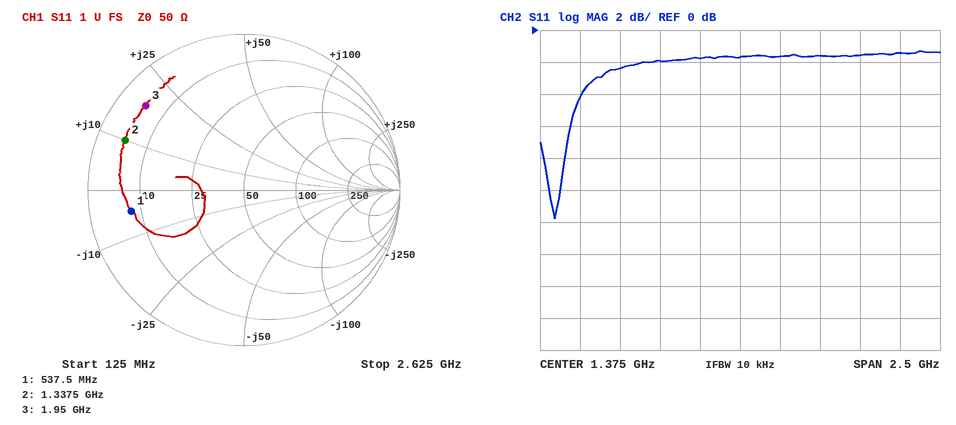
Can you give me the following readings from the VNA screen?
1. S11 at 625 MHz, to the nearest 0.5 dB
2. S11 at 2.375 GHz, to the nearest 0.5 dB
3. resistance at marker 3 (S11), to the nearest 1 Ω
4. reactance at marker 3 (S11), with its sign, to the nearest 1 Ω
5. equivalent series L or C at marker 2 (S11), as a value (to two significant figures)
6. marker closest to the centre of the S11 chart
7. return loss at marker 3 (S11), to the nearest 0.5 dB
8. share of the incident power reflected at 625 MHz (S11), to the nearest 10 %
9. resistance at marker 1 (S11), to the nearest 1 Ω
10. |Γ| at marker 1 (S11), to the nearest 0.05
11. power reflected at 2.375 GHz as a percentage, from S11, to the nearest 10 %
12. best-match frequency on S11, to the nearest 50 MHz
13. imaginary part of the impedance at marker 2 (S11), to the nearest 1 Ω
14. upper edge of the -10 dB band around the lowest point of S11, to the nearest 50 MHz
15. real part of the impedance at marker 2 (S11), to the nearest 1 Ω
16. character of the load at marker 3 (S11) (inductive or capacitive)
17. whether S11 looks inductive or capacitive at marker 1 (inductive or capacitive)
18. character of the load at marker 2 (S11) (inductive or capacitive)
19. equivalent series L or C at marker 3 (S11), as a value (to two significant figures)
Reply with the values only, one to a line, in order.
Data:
-2.5 dB
-1.5 dB
5 Ω
+18 Ω
1.2 nH
marker 1
1.5 dB
60 %
8 Ω
0.75
70 %
200 MHz
+10 Ω
250 MHz
5 Ω
inductive
capacitive
inductive
1.5 nH
